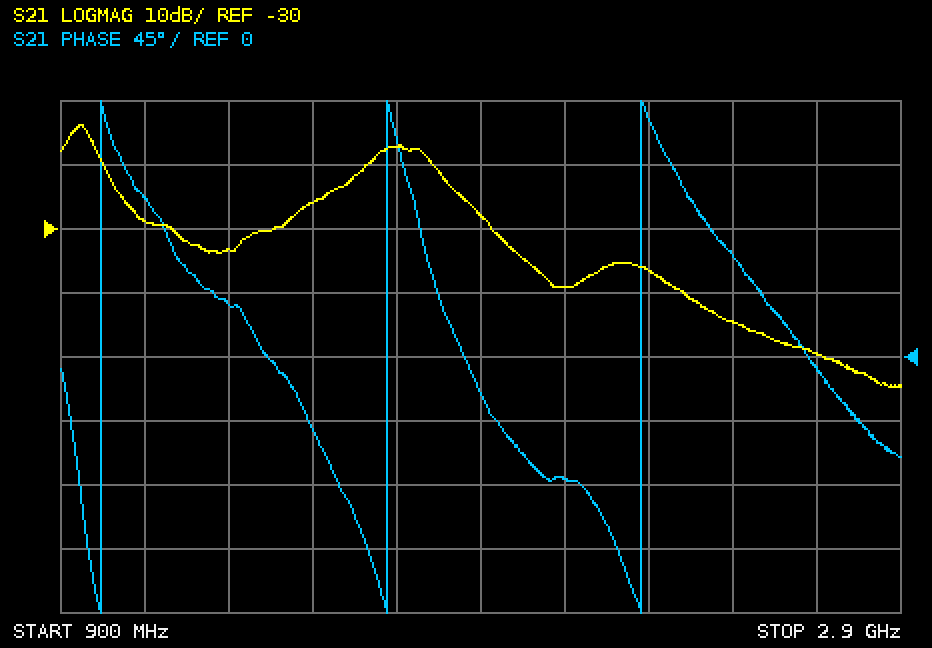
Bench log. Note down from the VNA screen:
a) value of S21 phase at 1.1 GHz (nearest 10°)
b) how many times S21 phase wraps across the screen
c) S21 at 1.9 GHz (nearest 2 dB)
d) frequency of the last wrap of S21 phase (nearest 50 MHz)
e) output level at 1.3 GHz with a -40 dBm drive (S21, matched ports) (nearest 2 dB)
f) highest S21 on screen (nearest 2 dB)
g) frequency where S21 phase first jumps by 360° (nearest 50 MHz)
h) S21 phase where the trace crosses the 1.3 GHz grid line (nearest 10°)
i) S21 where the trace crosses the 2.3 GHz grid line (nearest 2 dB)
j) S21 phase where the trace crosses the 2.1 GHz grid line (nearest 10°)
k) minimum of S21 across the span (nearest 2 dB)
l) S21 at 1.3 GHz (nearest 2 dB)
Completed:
110°
3
-28 dB
2.30 GHz
-74 dBm
-14 dB
1.00 GHz
40°
-36 dB
-90°
-54 dB
-34 dB
